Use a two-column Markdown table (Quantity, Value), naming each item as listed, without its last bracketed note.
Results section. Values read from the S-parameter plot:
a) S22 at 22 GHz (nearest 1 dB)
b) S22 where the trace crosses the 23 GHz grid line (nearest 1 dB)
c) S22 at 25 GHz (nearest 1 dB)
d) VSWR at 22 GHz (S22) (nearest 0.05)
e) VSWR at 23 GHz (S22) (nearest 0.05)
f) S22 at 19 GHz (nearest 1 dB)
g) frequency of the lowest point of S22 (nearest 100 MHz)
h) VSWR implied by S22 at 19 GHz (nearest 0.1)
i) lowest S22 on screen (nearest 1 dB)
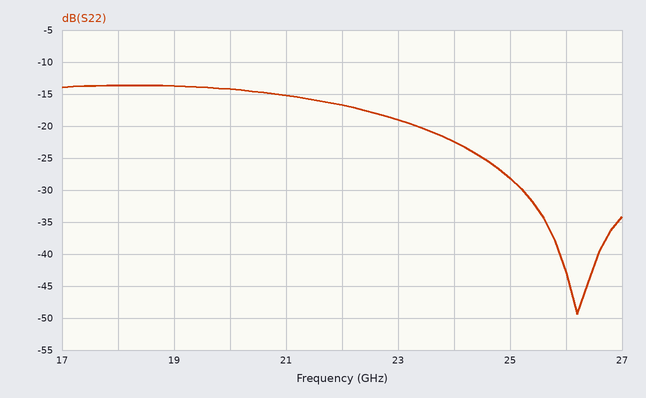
| Quantity | Value |
|---|---|
| S22 at 22 GHz | -17 dB |
| S22 where the trace crosses the 23 GHz grid line | -19 dB |
| S22 at 25 GHz | -28 dB |
| VSWR at 22 GHz (S22) | 1.35 |
| VSWR at 23 GHz (S22) | 1.25 |
| S22 at 19 GHz | -14 dB |
| frequency of the lowest point of S22 | 26.2 GHz |
| VSWR implied by S22 at 19 GHz | 1.5 |
| lowest S22 on screen | -49 dB |
